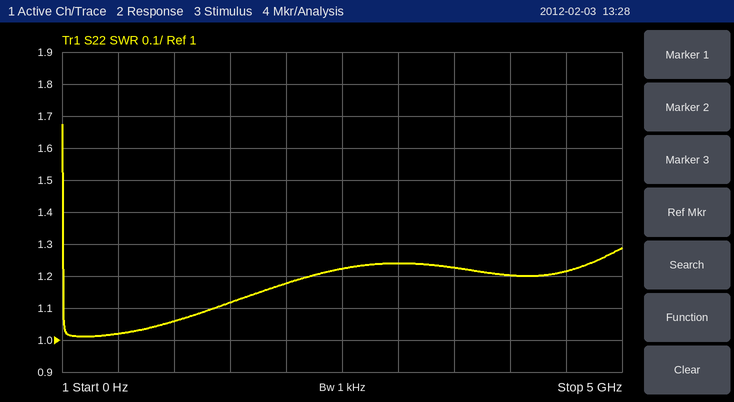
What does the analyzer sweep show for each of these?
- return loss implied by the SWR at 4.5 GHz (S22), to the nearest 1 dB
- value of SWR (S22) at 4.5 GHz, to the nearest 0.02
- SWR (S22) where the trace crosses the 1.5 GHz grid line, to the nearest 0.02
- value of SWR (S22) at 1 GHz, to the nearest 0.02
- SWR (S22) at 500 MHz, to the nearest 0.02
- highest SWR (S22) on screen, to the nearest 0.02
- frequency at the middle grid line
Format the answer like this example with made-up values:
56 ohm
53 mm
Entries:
20 dB
1.22
1.12
1.06
1.02
1.68
2.5 GHz
